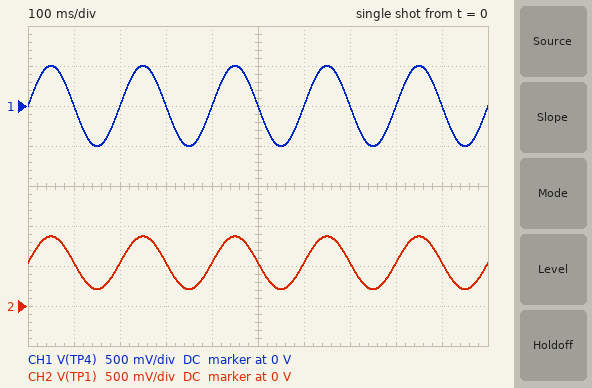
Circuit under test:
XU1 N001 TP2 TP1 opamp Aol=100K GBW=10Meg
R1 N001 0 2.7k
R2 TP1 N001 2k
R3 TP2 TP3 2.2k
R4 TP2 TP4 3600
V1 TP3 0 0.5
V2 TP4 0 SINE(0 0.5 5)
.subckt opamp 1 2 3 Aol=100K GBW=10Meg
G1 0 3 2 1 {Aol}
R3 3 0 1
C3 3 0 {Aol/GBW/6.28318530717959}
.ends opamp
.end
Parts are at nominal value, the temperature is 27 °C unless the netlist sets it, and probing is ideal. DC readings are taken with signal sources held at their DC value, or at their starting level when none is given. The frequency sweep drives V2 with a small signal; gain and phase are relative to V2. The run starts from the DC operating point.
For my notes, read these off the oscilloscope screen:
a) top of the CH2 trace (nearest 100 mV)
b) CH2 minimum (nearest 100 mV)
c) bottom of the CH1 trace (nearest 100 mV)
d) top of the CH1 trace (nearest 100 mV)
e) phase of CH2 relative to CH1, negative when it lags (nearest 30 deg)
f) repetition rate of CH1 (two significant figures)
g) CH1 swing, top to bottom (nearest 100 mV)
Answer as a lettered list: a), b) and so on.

a) 900 mV
b) 200 mV
c) -500 mV
d) 500 mV
e) 0 deg
f) 5.0 Hz
g) 1.0 V
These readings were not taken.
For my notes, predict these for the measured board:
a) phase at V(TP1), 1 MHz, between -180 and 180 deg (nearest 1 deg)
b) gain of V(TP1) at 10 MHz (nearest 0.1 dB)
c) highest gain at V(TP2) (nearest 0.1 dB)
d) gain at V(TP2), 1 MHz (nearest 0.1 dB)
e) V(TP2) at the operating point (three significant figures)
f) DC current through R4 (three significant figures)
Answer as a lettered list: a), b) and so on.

a) -10 deg
b) -9.7 dB
c) -8.4 dB
d) -8.4 dB
e) 310 mV
f) 86.2 µA
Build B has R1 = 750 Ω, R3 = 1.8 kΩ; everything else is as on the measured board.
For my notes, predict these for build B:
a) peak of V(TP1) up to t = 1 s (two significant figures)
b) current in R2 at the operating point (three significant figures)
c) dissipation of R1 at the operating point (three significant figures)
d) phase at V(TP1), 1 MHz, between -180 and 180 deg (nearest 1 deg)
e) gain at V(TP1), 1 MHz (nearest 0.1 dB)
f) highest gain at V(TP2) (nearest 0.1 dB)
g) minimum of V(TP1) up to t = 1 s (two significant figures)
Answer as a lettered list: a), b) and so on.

a) 1.8 V
b) 444 µA
c) 148 µW
d) -20 deg
e) 1.2 dB
f) -9.5 dB
g) 610 mV
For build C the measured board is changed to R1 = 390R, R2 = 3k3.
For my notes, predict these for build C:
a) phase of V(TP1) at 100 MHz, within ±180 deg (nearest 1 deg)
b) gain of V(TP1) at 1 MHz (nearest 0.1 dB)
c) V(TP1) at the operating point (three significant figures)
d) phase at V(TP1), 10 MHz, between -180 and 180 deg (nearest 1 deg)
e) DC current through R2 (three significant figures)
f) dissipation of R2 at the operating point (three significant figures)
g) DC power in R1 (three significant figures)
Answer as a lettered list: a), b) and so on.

a) -89 deg
b) 8.3 dB
c) 2.94 V
d) -84 deg
e) 796 µA
f) 2.09 mW
g) 247 µW
